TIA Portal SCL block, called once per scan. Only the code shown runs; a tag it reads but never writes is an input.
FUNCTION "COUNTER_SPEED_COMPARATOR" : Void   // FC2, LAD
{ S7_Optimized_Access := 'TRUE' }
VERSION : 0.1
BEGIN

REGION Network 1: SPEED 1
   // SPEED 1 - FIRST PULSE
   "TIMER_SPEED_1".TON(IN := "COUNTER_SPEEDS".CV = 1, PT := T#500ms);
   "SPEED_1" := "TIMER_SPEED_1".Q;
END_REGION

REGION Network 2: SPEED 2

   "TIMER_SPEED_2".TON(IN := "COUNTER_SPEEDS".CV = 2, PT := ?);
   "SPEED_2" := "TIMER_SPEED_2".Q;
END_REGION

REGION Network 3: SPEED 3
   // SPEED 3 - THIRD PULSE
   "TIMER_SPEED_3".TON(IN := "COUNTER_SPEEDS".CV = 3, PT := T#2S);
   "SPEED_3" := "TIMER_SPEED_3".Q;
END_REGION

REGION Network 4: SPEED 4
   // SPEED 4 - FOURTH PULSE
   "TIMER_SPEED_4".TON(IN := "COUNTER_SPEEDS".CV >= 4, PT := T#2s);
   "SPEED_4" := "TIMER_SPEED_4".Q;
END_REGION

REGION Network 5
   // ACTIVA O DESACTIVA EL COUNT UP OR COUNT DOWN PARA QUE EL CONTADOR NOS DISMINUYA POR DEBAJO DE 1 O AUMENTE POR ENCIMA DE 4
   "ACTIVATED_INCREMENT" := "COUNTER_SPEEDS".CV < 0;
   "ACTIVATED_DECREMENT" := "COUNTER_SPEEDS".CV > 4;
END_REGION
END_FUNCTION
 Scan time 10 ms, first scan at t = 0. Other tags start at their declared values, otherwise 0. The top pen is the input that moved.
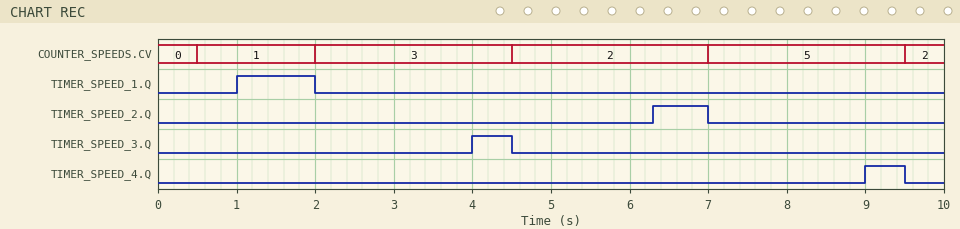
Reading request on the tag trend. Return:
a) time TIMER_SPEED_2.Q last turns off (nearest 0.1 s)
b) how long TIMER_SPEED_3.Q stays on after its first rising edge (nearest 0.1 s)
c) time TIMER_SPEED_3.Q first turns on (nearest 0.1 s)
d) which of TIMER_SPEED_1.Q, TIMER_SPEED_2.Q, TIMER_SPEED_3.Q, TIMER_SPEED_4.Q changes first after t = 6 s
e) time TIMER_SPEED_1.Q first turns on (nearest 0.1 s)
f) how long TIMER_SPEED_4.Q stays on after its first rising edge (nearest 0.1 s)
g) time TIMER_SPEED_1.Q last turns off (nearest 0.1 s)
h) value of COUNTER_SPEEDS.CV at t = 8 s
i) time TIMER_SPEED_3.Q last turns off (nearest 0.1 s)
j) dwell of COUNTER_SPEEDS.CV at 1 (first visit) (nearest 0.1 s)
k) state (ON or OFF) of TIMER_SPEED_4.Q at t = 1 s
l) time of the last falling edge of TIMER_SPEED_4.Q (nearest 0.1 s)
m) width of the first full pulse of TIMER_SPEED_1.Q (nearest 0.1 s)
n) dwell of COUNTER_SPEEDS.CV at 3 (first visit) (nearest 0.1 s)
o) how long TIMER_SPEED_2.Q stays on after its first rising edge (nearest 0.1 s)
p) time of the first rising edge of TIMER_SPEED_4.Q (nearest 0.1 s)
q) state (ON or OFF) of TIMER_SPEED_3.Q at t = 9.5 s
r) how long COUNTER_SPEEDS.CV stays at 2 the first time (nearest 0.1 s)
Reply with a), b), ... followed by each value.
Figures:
a) 7.0 s
b) 0.5 s
c) 4.0 s
d) TIMER_SPEED_2.Q
e) 1.0 s
f) 0.5 s
g) 2.0 s
h) 5
i) 4.5 s
j) 1.5 s
k) OFF
l) 9.5 s
m) 1.0 s
n) 2.5 s
o) 0.7 s
p) 9.0 s
q) OFF
r) 2.5 s
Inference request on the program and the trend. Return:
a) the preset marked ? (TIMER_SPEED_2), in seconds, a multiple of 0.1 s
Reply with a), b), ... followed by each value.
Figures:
a) 1.8 s
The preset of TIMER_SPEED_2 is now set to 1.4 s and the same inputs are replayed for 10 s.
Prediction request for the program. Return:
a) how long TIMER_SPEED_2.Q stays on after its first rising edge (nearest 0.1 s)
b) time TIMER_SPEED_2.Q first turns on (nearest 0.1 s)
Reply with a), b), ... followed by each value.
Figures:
a) 1.1 s
b) 5.9 s
